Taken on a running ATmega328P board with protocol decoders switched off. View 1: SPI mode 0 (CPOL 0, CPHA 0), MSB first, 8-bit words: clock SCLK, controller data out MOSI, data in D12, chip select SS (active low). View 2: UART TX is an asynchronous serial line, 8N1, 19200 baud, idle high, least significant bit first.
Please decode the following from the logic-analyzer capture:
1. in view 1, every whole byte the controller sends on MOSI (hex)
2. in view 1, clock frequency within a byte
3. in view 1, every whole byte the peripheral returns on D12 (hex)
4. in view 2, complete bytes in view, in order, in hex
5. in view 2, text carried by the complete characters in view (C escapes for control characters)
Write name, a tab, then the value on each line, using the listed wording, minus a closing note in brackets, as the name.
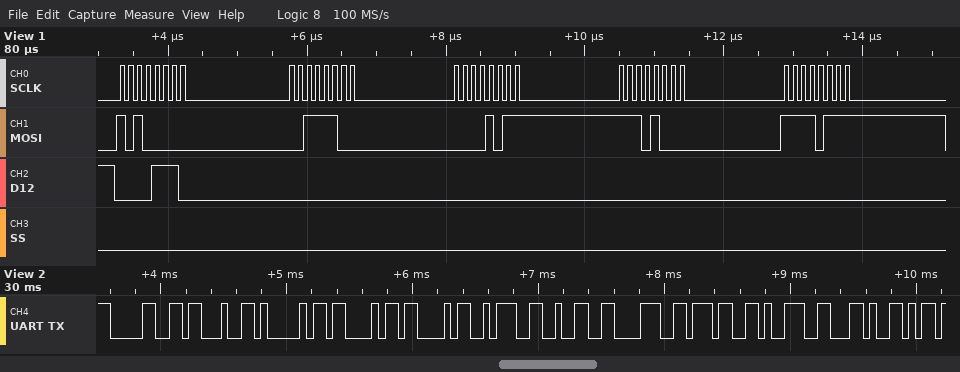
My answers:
in view 1, every whole byte the controller sends on MOSI	0xA0 0x3C 0x0B 0xE8 0xF7
in view 1, clock frequency within a byte	8 MHz
in view 1, every whole byte the peripheral returns on D12	0x0E 0x00 0x00 0x00 0x00
in view 2, complete bytes in view, in order, in hex	0x30 0x23 0x41 0x43 0x43 0x3A 0x32 0x38 0x37 0x39 0x2C
in view 2, text carried by the complete characters in view	"0#ACC:2879,"
